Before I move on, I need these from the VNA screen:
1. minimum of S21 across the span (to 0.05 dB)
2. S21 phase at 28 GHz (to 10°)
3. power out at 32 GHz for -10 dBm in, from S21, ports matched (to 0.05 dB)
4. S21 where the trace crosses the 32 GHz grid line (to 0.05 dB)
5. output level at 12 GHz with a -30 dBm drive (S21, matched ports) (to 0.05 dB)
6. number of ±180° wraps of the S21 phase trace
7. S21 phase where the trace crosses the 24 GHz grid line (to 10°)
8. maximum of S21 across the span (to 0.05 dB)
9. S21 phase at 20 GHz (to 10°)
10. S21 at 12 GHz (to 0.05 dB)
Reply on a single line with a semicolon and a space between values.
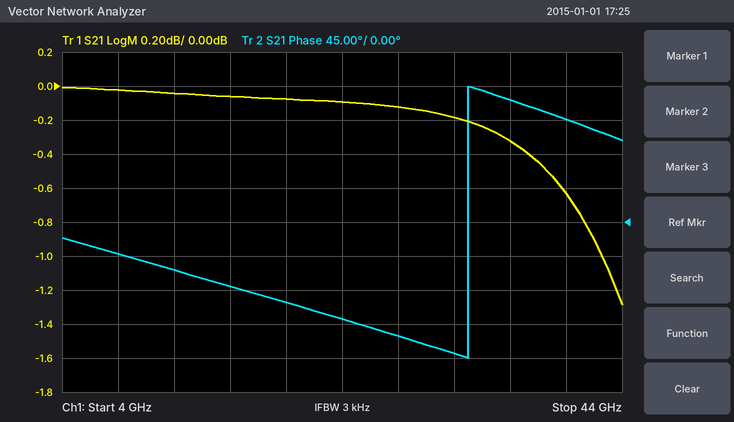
-1.30 dB; -150°; -10.20 dBm; -0.20 dB; -30.05 dBm; 1; -130°; 0.00 dB; -110°; -0.05 dB
